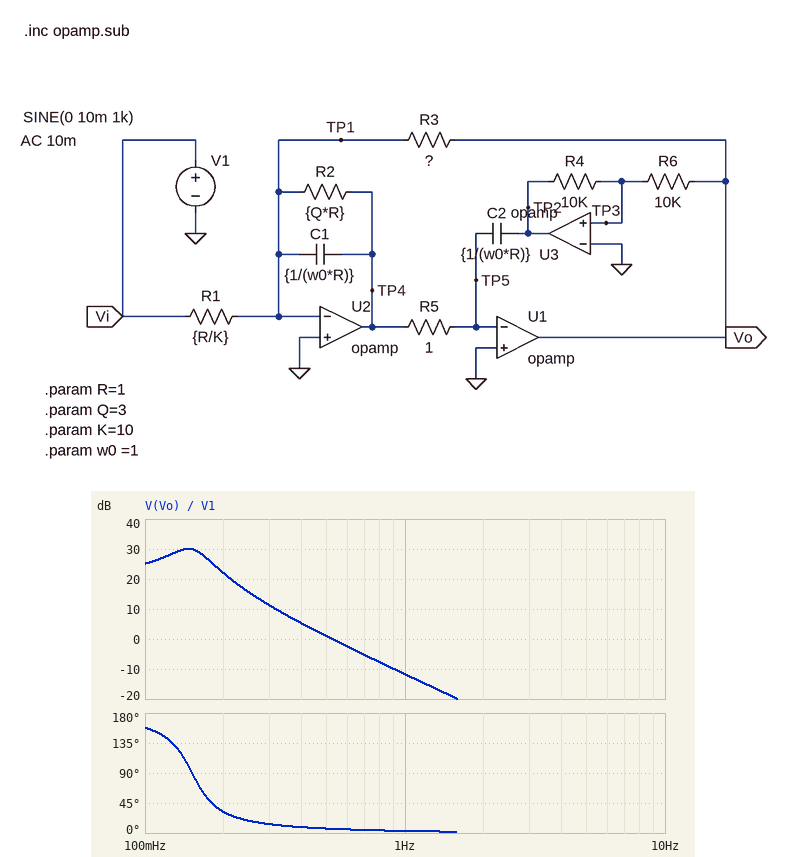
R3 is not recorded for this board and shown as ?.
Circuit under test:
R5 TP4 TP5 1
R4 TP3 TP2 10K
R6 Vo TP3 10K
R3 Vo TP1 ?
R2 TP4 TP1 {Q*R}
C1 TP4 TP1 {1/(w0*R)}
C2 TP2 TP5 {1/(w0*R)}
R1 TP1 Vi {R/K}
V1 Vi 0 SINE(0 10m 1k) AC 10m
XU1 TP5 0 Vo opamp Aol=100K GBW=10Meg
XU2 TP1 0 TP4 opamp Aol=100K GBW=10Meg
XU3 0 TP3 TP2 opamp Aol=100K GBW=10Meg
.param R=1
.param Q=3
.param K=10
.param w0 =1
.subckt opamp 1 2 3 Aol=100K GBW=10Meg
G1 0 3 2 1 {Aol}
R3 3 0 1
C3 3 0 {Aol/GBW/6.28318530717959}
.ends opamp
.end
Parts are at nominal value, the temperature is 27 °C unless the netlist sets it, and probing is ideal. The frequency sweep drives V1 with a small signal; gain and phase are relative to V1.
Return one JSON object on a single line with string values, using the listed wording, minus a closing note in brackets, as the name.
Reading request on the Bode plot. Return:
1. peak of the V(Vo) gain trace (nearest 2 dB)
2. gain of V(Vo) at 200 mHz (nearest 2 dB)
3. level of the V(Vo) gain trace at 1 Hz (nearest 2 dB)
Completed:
{"peak of the V(Vo) gain trace": "30 dB", "gain of V(Vo) at 200 mHz": "22 dB", "level of the V(Vo) gain trace at 1 Hz": "-12 dB"}
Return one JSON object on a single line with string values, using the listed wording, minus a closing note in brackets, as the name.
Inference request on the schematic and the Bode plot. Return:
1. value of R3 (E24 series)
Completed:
{"value of R3": "1.1 Ω"}
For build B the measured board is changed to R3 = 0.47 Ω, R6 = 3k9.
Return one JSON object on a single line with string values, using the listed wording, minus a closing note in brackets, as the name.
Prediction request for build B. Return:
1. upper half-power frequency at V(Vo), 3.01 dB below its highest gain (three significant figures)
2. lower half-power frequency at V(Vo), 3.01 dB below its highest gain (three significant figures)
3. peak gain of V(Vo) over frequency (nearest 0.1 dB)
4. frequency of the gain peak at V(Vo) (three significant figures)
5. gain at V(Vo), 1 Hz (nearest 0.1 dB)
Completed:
{"upper half-power frequency at V(Vo), 3.01 dB below its highest gain": "165 mHz", "lower half-power frequency at V(Vo), 3.01 dB below its highest gain": "110 mHz", "peak gain of V(Vo) over frequency": "22.3 dB", "frequency of the gain peak at V(Vo)": "140 mHz", "gain at V(Vo), 1 Hz": "-19.9 dB"}
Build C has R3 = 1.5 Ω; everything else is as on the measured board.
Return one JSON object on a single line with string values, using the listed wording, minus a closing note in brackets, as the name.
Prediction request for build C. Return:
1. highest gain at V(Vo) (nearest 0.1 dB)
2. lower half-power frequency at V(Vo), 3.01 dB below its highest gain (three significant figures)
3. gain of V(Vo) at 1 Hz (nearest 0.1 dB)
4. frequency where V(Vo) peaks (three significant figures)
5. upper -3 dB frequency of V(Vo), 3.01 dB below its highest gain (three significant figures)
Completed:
{"highest gain at V(Vo)": "31.5 dB", "lower half-power frequency at V(Vo), 3.01 dB below its highest gain": "93.4 mHz", "gain of V(Vo) at 1 Hz": "-11.8 dB", "frequency where V(Vo) peaks": "124 mHz", "upper -3 dB frequency of V(Vo), 3.01 dB below its highest gain": "149 mHz"}
